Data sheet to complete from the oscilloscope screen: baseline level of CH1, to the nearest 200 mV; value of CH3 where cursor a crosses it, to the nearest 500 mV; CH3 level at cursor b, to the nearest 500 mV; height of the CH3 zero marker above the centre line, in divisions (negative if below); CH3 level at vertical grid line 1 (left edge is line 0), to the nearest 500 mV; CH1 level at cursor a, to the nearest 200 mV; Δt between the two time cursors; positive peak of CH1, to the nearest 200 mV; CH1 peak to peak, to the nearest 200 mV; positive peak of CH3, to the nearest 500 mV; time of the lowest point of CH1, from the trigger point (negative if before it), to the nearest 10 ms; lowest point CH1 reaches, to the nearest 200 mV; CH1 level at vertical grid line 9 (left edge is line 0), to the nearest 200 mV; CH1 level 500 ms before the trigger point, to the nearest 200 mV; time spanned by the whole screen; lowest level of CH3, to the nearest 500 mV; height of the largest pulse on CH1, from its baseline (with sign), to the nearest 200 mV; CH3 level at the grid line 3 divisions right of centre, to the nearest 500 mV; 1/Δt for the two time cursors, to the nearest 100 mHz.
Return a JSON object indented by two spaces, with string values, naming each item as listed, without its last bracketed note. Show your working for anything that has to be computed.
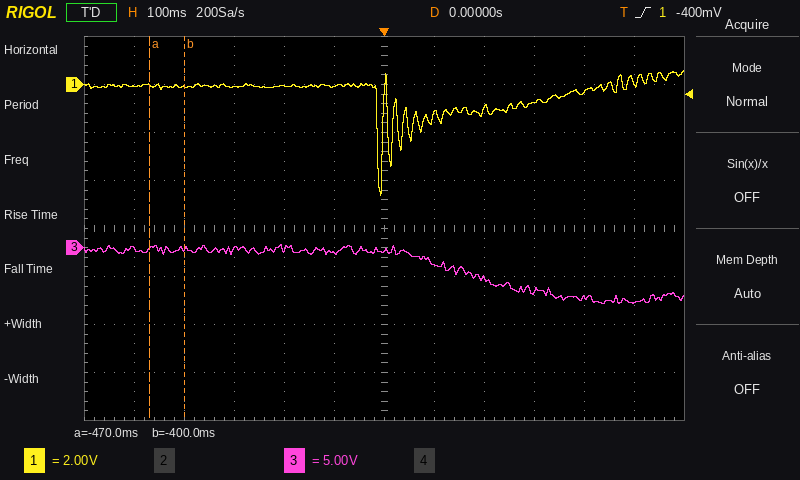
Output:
{
  "baseline level of CH1, to the nearest 200 mV": "0.0 V",
  "value of CH3 where cursor a crosses it, to the nearest 500 mV": "0.0 V",
  "CH3 level at cursor b, to the nearest 500 mV": "0.0 V",
  "height of the CH3 zero marker above the centre line, in divisions": "-0.4 div",
  "CH3 level at vertical grid line 1 (left edge is line 0), to the nearest 500 mV": "0.0 V",
  "CH1 level at cursor a, to the nearest 200 mV": "0.0 V",
  "Δt between the two time cursors": "-400 ms − (-470 ms) = 70 ms",
  "positive peak of CH1, to the nearest 200 mV": "600 mV",
  "CH1 peak to peak, to the nearest 200 mV": "600 mV − (-4.6 V) = 5.2 V",
  "positive peak of CH3, to the nearest 500 mV": "500 mV",
  "time of the lowest point of CH1, from the trigger point (negative if before it), to the nearest 10 ms": "-10 ms",
  "lowest point CH1 reaches, to the nearest 200 mV": "-4.6 V",
  "CH1 level at vertical grid line 9 (left edge is line 0), to the nearest 200 mV": "-800 mV",
  "CH1 level 500 ms before the trigger point, to the nearest 200 mV": "0.0 V",
  "time spanned by the whole screen": "1.2 s",
  "lowest level of CH3, to the nearest 500 mV": "-6.0 V",
  "height of the largest pulse on CH1, from its baseline (with sign), to the nearest 200 mV": "-4.6 V − (0.0 V) = -4.6 V",
  "CH3 level at the grid line 3 divisions right of centre, to the nearest 500 mV": "-4.5 V",
  "1/Δt for the two time cursors, to the nearest 100 mHz": "1 / 70 ms ≈ 14.3 Hz"
}
